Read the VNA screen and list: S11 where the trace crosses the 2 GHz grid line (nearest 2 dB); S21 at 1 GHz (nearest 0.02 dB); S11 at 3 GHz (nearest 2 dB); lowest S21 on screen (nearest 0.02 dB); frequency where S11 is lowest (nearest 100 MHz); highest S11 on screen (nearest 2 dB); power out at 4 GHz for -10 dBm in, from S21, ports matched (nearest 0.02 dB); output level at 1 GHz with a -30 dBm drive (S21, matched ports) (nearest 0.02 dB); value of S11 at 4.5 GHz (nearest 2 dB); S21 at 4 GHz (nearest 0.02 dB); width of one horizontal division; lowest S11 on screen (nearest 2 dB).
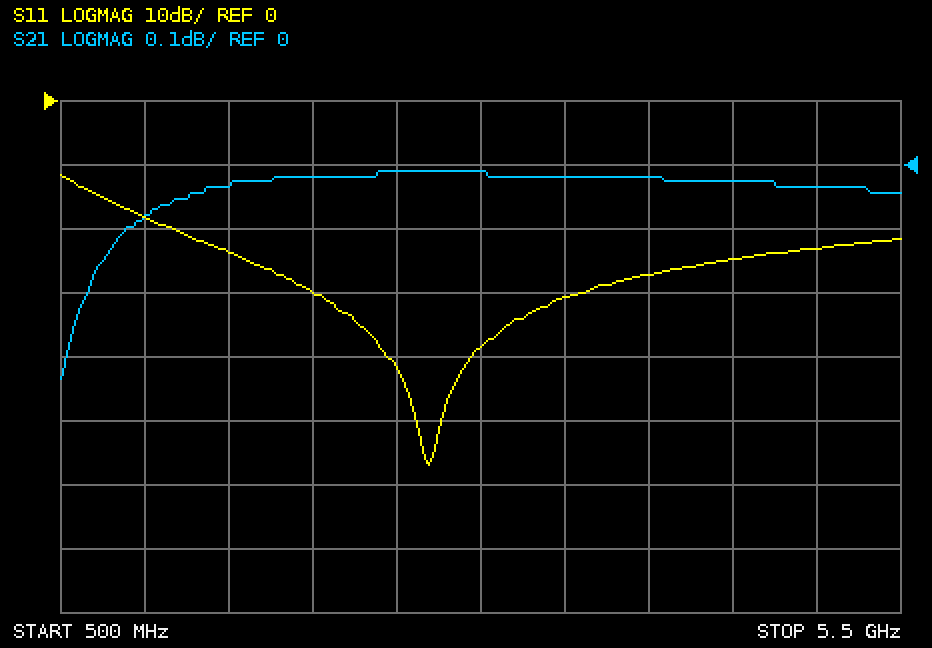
-30 dB
-0.08 dB
-38 dB
-0.34 dB
2.7 GHz
-12 dB
-10.02 dBm
-30.08 dBm
-24 dB
-0.02 dB
500 MHz
-56 dB
